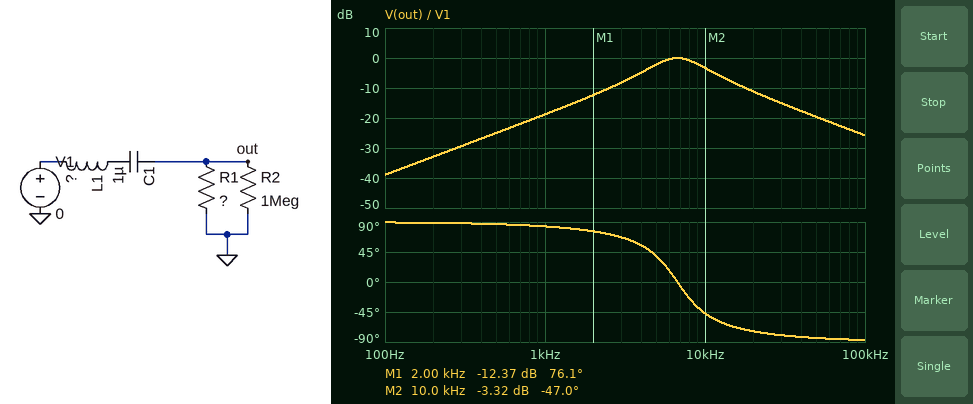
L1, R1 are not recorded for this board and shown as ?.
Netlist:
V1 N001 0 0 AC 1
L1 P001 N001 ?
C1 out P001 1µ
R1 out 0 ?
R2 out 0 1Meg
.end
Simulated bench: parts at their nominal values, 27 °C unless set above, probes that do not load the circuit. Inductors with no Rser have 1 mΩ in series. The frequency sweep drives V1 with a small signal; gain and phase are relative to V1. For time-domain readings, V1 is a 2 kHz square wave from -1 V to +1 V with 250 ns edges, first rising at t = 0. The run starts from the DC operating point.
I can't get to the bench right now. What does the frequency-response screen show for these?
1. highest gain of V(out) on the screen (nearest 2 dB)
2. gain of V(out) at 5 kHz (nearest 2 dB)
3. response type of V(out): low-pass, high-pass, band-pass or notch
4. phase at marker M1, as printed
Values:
0 dB
-2 dB
band-pass
76.1 deg
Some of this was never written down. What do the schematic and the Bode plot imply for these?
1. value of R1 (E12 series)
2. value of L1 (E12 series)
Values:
18 Ω
560 µH
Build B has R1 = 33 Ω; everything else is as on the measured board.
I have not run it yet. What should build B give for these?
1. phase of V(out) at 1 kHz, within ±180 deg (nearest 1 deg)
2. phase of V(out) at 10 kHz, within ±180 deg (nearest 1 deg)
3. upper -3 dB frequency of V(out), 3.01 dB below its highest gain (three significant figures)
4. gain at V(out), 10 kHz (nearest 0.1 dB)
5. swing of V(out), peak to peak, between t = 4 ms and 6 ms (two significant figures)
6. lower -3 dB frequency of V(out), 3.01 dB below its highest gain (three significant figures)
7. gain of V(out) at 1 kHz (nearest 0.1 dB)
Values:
78 deg
-30 deg
12.9 kHz
-1.3 dB
2.6 V
3.51 kHz
-13.7 dB
